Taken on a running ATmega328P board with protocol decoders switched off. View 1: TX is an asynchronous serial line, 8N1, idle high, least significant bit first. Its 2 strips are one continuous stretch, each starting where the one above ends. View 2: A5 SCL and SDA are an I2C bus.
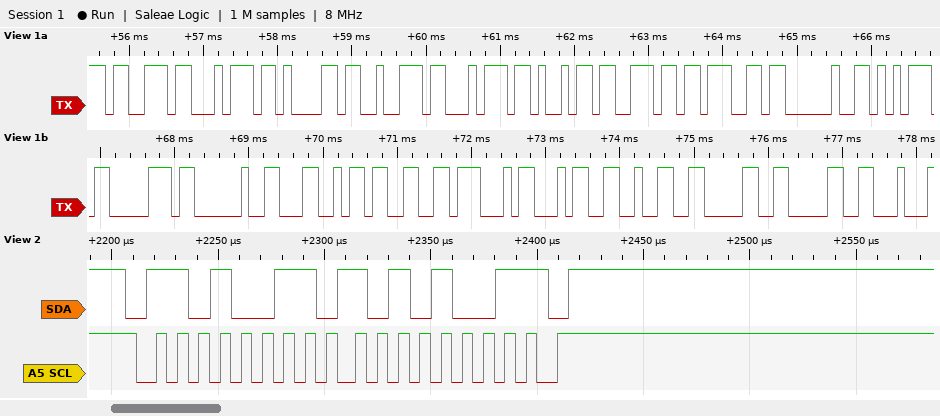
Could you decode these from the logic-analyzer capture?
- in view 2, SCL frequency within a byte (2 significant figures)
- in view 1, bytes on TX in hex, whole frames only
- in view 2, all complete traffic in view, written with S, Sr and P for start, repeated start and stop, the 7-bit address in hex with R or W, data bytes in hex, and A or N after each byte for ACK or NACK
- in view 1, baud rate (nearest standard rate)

100 kHz
73 74 61 72 74 69 6E 67 20 75 70 20 4C 33 47 34 32 30 30
S 69R A A9 N P
9600 baud
